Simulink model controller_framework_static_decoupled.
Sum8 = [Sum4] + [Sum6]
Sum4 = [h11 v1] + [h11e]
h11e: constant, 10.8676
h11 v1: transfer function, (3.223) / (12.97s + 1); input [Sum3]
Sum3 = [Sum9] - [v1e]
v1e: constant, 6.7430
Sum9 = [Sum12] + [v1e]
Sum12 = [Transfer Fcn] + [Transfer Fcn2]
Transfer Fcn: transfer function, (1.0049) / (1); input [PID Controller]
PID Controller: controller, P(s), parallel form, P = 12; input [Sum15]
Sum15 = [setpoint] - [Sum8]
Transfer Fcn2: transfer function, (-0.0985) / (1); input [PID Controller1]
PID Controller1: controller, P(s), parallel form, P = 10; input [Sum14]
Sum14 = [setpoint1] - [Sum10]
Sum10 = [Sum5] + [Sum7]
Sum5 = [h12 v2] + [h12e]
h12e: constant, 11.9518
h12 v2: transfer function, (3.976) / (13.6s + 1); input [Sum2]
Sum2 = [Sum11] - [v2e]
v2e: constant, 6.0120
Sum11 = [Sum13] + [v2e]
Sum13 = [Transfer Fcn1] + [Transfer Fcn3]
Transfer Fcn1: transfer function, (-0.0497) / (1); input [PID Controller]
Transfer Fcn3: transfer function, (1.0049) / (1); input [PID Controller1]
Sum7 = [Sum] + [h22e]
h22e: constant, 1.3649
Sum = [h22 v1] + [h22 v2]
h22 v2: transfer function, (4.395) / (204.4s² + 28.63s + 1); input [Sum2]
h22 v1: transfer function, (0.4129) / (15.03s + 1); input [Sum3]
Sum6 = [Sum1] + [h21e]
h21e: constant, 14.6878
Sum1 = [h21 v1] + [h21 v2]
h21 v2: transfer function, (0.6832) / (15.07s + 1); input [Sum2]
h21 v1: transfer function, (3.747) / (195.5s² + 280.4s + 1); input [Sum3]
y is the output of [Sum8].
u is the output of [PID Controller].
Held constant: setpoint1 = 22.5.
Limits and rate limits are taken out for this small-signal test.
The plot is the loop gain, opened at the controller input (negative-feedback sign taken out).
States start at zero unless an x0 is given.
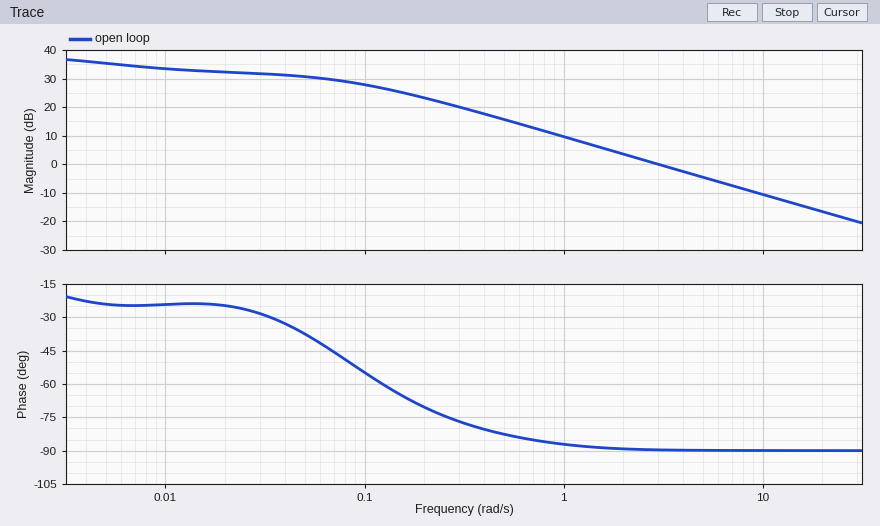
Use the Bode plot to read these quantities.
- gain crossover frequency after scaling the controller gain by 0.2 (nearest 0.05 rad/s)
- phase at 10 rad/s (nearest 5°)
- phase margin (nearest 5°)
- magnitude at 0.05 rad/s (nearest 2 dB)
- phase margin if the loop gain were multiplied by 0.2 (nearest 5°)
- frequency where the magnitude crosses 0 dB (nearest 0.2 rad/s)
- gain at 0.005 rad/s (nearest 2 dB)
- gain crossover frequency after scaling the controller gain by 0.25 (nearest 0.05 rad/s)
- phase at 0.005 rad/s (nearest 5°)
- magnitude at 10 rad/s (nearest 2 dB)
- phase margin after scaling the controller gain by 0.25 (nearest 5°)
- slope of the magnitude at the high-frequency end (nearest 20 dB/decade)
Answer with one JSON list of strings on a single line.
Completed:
["0.60 rad/s", "-90°", "90°", "30 dB", "95°", "3.0 rad/s", "36 dB", "0.75 rad/s", "-25°", "-10 dB", "95°", "-20 dB/decade"]
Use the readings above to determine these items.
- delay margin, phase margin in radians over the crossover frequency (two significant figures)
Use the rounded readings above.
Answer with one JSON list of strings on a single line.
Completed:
["0.52 s"]
